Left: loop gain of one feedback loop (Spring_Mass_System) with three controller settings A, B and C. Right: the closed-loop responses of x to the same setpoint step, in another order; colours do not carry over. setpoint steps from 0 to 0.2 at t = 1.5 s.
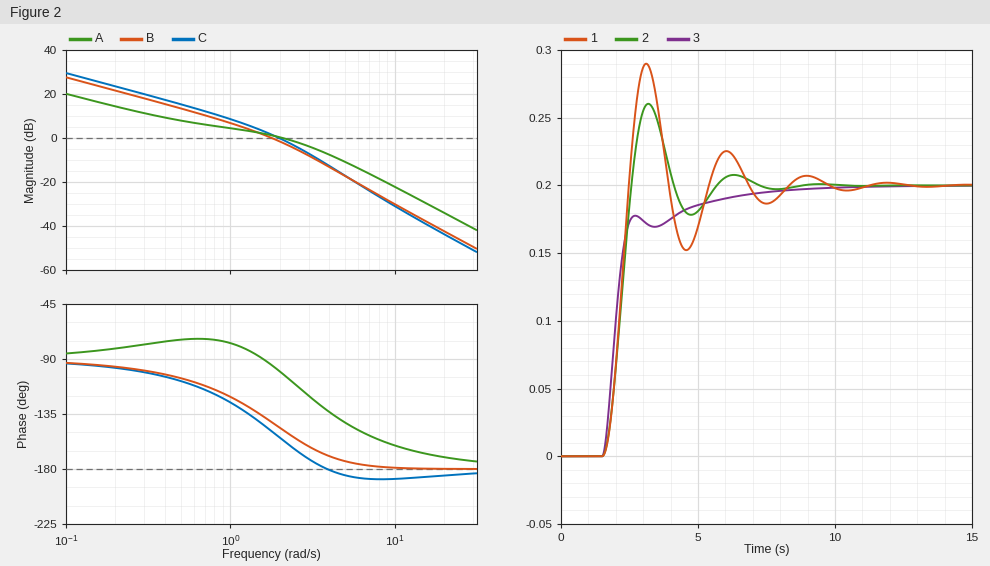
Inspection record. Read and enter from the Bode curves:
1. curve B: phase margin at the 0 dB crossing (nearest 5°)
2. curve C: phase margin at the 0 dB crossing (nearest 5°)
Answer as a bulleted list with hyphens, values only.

- 40°
- 25°
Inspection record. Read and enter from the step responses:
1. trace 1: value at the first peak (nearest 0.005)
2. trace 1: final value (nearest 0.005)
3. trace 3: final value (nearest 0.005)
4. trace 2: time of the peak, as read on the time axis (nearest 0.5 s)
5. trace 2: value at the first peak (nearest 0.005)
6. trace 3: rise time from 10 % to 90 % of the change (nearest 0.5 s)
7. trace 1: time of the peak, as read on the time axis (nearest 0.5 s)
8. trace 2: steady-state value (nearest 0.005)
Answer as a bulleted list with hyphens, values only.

- 0.290
- 0.200
- 0.200
- 3.0 s
- 0.260
- 2.5 s
- 3.0 s
- 0.200
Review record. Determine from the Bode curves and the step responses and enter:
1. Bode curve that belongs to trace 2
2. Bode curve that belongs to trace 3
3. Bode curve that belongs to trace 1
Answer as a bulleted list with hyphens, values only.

- B
- A
- C
